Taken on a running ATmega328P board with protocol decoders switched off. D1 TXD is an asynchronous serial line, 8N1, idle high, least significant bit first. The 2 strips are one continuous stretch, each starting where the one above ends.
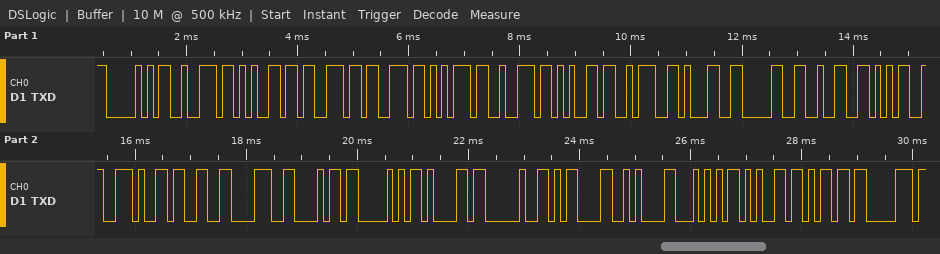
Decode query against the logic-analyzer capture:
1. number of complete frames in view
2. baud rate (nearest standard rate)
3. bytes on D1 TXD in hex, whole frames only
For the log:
26
9600 baud
50 72 65 73 73 75 72 65 3A 31 30 32 35 2E 33 38 68 50 61 20 0D 0A 54 65 6D 70
